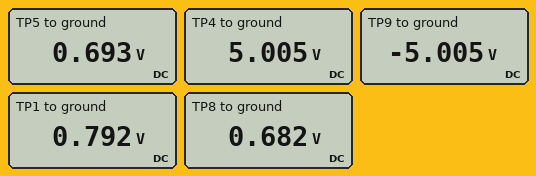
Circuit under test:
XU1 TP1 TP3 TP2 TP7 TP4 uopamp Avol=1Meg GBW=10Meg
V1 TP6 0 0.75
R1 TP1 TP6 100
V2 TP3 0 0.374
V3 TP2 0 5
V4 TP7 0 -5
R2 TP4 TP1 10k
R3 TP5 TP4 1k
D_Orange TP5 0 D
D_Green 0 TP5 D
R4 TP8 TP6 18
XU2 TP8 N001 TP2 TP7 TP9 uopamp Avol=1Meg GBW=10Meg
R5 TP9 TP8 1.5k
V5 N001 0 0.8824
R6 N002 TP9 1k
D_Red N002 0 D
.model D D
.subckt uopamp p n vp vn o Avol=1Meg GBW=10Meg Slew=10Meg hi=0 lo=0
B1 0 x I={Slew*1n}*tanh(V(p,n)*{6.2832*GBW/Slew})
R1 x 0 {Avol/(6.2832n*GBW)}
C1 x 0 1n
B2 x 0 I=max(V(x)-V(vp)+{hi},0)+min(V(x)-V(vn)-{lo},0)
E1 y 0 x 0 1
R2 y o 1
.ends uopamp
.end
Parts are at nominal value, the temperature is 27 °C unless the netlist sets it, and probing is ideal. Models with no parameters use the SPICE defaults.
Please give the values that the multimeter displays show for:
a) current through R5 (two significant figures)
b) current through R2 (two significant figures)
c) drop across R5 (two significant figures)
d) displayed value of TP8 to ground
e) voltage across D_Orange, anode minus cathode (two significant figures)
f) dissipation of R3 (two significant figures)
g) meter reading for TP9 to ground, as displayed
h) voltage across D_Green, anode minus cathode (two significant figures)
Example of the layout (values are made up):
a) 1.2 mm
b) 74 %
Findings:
a) 3.8 mA
b) 420 µA
c) 5.7 V
d) 0.682 V
e) 690 mV
f) 19 mW
g) -5.005 V
h) -690 mV
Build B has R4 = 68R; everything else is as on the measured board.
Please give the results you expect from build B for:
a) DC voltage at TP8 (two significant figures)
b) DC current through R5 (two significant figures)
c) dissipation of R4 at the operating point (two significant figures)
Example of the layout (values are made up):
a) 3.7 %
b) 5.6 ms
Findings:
a) 500 mV
b) 3.7 mA
c) 920 µW
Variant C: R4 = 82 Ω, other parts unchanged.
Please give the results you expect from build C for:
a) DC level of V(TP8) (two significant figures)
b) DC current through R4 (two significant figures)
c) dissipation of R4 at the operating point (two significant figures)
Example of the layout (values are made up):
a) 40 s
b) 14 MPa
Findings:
a) 450 mV
b) 3.6 mA
c) 1.1 mW
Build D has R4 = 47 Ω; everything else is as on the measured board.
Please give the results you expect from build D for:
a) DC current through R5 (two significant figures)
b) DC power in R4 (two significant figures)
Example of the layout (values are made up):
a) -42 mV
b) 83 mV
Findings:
a) 3.7 mA
b) 650 µW
